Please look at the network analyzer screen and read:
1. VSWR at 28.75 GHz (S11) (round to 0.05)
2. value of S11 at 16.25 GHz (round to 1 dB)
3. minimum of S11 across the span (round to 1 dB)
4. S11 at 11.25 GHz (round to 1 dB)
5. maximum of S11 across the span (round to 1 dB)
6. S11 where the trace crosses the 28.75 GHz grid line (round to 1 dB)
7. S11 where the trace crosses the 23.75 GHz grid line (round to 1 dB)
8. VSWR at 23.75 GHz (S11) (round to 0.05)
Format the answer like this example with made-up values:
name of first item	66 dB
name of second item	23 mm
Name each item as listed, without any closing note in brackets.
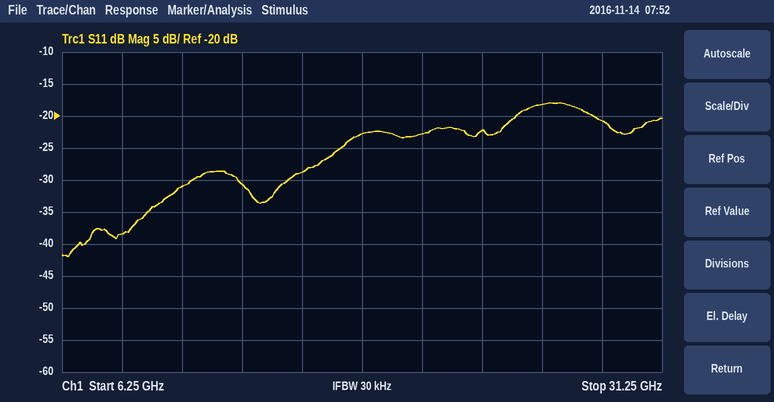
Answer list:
VSWR at 28.75 GHz (S11)	1.20
value of S11 at 16.25 GHz	-29 dB
minimum of S11 across the span	-42 dB
S11 at 11.25 GHz	-31 dB
maximum of S11 across the span	-18 dB
S11 where the trace crosses the 28.75 GHz grid line	-21 dB
S11 where the trace crosses the 23.75 GHz grid line	-22 dB
VSWR at 23.75 GHz (S11)	1.15
